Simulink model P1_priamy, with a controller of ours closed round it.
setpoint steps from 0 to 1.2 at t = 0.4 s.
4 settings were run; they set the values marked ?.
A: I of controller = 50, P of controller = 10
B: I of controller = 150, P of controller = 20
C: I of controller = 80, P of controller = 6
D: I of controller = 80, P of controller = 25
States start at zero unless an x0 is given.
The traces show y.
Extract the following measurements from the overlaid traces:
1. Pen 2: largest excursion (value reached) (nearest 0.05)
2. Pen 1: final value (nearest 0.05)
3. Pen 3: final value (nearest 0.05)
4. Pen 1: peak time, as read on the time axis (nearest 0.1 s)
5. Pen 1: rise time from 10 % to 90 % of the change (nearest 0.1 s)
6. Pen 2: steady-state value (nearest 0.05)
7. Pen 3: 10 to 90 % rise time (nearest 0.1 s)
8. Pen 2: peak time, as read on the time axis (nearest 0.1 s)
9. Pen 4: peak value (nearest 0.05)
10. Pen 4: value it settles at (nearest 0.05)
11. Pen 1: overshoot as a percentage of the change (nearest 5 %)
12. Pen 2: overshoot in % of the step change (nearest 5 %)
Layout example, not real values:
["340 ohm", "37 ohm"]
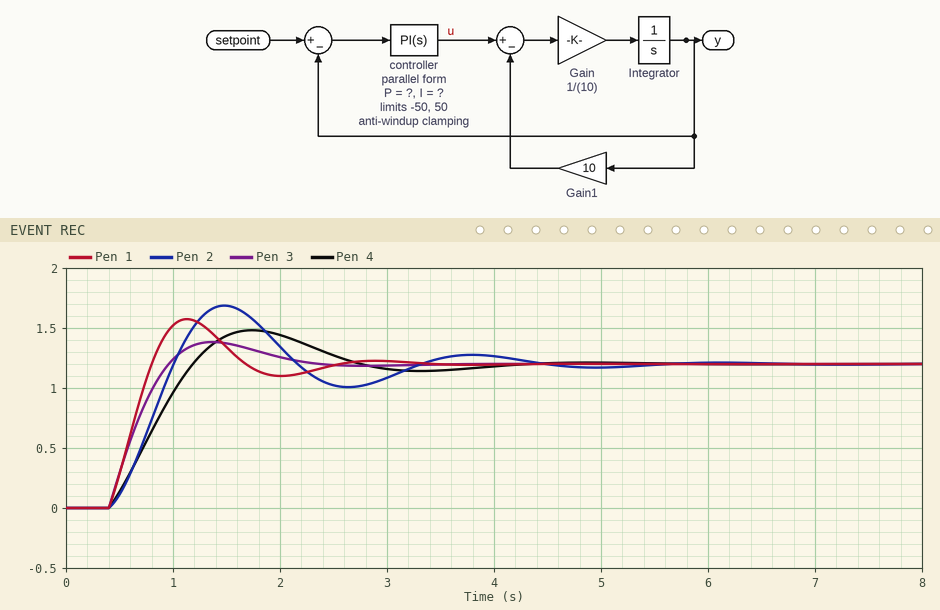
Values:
["1.70", "1.20", "1.20", "1.1 s", "0.3 s", "1.20", "0.4 s", "1.5 s", "1.50", "1.20", "30 %", "40 %"]
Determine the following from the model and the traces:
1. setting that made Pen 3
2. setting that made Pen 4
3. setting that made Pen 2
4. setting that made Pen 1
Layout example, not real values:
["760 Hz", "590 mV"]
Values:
["D", "A", "C", "B"]
